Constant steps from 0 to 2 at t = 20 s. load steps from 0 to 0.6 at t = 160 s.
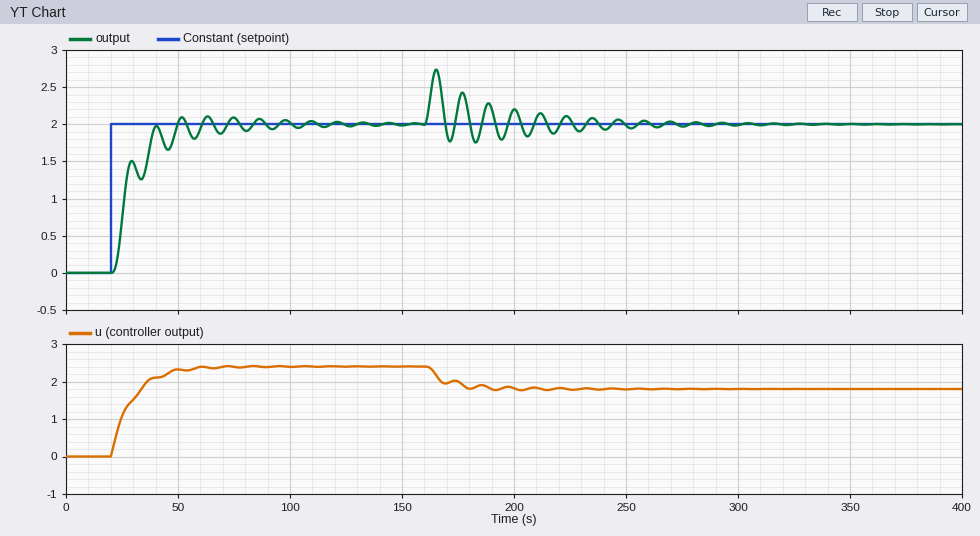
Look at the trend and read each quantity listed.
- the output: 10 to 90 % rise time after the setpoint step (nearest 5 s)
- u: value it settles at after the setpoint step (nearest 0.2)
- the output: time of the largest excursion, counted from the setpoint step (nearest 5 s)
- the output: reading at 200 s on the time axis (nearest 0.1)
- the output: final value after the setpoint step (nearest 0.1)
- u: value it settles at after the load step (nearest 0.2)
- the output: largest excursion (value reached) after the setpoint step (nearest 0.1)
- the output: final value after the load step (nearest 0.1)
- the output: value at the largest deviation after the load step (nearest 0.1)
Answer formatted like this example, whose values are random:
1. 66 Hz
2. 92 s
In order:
1. 15 s
2. 2.4
3. 45 s
4. 2.2
5. 2.0
6. 1.8
7. 2.1
8. 2.0
9. 2.7
